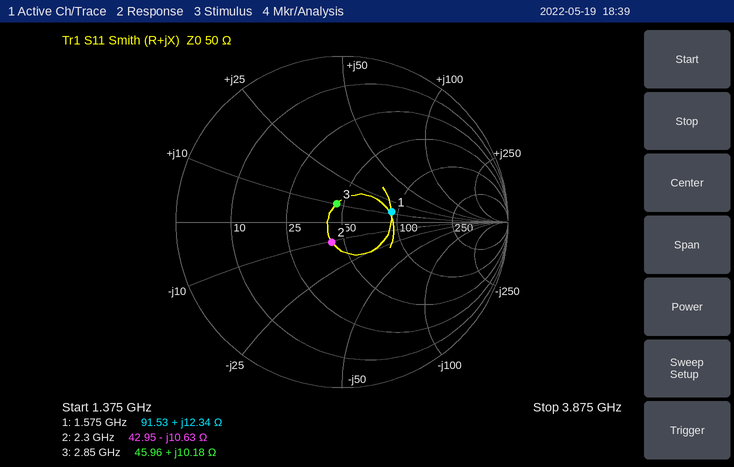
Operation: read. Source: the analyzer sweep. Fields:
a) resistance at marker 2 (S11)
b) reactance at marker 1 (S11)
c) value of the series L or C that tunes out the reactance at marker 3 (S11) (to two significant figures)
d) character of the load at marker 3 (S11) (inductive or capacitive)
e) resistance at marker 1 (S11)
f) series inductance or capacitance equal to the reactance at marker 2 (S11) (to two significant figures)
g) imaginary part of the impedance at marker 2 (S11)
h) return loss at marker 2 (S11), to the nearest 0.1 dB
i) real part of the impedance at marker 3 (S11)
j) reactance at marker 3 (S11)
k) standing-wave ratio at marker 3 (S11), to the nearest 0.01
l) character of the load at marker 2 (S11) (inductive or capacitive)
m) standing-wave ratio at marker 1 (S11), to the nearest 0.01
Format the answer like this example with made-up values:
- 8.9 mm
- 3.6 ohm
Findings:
- 42.95 Ω
- +12.34 Ω
- 5.5 pF
- inductive
- 91.53 Ω
- 6.5 pF
- -10.63 Ω
- 17.3 dB
- 45.96 Ω
- +10.18 Ω
- 1.26
- capacitive
- 1.88
